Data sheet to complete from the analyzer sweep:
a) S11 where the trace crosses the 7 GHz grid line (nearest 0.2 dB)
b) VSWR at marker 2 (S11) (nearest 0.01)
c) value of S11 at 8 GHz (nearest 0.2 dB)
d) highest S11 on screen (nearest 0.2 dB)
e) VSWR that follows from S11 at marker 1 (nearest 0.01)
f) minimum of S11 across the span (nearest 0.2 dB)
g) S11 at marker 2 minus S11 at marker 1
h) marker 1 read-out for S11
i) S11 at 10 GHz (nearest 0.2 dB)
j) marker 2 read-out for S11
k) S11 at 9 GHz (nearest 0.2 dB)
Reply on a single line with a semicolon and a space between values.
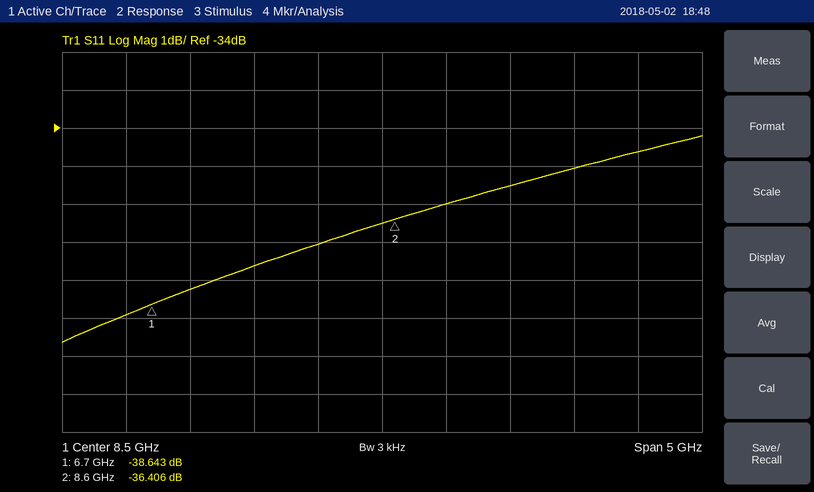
-38.2 dB; 1.03; -37.0 dB; -34.2 dB; 1.02; -39.6 dB; 2.237 dB; -38.643 dB; -35.0 dB; -36.406 dB; -36.0 dB
